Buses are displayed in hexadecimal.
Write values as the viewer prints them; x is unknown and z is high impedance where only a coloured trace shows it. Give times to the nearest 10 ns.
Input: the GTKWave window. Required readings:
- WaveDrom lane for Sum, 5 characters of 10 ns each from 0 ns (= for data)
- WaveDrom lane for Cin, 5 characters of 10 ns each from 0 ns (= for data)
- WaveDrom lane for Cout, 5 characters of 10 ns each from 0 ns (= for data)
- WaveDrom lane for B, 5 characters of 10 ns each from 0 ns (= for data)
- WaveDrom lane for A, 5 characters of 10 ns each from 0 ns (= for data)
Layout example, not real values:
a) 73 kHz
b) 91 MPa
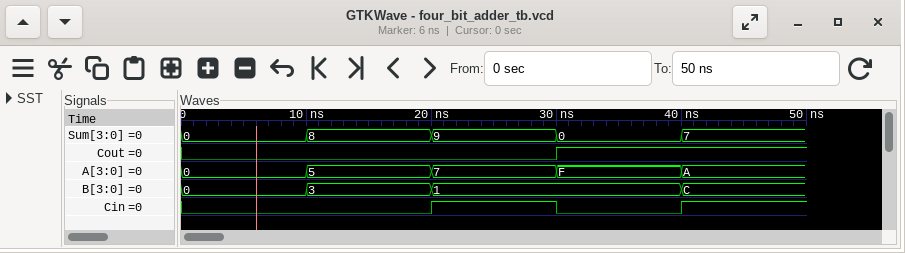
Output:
a) {name: 'Sum', wave: '=====', data: '0 8 9 0 7'}
b) {name: 'Cin', wave: '0.101'}
c) {name: 'Cout', wave: '0..1.'}
d) {name: 'B', wave: '===.=', data: '0 3 1 C'}
e) {name: 'A', wave: '=====', data: '0 5 7 F A'}
